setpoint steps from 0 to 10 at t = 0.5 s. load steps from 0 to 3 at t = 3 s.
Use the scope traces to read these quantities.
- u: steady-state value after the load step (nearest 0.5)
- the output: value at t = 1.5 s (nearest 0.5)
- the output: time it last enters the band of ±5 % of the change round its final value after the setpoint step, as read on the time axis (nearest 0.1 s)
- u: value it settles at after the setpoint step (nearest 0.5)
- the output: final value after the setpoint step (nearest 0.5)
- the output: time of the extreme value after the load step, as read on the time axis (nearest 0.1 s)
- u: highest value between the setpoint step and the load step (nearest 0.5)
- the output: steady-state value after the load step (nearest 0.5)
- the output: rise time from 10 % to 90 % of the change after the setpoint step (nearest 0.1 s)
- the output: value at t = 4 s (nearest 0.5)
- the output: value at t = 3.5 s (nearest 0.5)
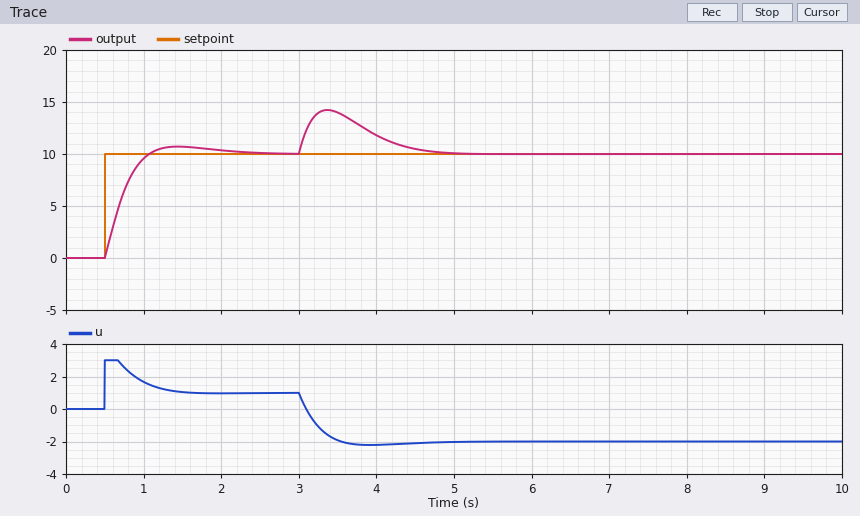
-2.0
10.5
1.8 s
1.0
10.0
3.4 s
3.0
10.0
0.4 s
12.0
14.0
